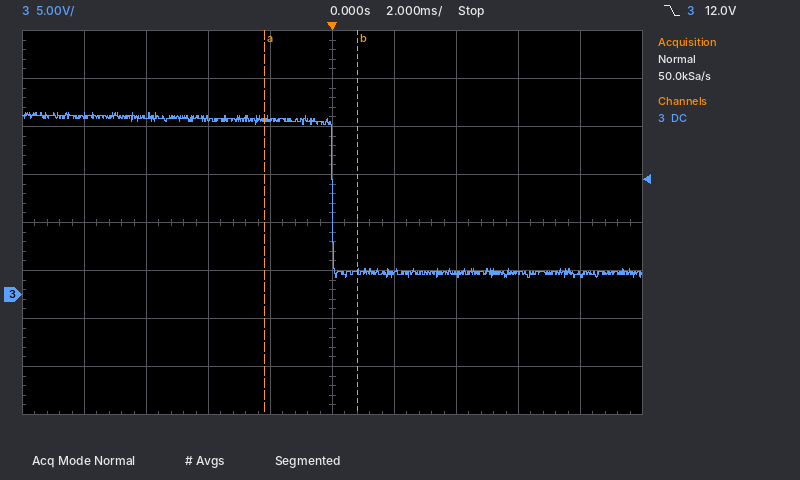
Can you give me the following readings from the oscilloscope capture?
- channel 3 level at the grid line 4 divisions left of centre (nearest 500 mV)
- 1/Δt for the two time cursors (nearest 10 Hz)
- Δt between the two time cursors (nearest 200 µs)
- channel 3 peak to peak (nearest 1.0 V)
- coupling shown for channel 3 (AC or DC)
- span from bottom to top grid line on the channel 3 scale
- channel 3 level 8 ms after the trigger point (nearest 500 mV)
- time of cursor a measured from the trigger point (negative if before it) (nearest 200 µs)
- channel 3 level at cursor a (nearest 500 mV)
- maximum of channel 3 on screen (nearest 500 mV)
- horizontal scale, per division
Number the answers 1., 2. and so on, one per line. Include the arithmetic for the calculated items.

1. 18.5 V
2. 1 / 3.0 ms ≈ 330 Hz
3. 3.0 ms
4. 17.0 V
5. DC
6. 40 V
7. 2.0 V
8. -2.2 ms
9. 18.5 V
10. 19.0 V
11. 2 ms
